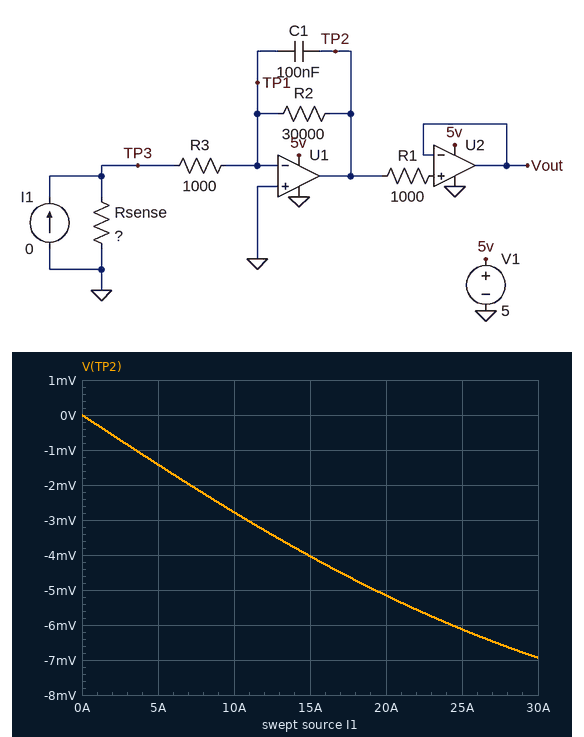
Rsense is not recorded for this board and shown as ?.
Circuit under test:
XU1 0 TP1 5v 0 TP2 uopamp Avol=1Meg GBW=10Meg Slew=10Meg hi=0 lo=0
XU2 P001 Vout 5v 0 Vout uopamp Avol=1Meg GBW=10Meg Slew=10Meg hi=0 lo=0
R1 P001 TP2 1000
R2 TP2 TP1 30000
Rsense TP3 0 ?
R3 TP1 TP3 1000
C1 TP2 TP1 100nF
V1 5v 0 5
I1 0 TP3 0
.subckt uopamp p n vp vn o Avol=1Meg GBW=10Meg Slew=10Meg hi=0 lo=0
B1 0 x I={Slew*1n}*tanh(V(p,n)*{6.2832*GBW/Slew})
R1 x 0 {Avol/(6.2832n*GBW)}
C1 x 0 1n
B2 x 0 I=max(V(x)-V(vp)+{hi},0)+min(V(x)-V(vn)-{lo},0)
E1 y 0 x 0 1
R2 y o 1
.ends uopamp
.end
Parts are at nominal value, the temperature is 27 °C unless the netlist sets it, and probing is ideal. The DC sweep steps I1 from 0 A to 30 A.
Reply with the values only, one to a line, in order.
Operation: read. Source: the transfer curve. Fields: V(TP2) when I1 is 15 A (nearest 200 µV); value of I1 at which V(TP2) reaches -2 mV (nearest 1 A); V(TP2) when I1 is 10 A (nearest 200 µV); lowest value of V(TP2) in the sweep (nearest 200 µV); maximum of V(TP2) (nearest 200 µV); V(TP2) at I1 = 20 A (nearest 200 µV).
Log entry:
-4.0 mV
7 A
-2.8 mV
-7.0 mV
0 V
-5.2 mV
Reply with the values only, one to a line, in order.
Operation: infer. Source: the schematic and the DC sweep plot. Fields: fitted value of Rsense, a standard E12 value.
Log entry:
4.7 mΩ
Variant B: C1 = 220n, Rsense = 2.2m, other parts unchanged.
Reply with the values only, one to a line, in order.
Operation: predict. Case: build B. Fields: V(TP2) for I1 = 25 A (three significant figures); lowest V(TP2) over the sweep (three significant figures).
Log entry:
-3.22 mV
-3.80 mV
